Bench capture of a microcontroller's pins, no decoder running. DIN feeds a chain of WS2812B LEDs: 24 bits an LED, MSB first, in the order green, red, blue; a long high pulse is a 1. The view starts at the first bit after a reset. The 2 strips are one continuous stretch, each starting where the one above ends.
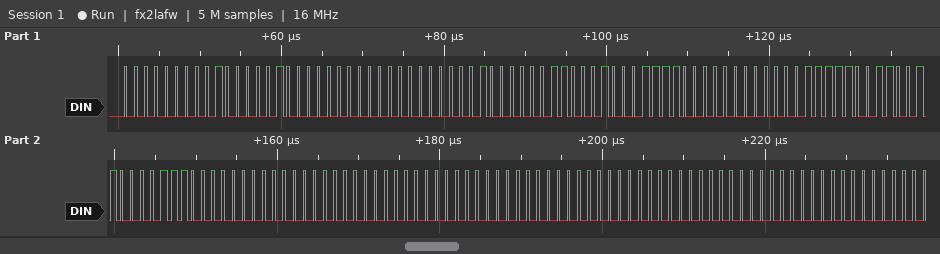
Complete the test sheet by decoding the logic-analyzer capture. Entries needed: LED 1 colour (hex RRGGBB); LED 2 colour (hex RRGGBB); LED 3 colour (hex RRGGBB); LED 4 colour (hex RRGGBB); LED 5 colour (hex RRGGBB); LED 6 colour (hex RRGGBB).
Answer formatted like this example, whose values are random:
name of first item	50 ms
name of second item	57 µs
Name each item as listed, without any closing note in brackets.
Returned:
LED 1 colour	#410000
LED 2 colour	#100031
LED 3 colour	#001E1F
LED 4 colour	#0E3300
LED 5 colour	#000000
LED 6 colour	#000000
